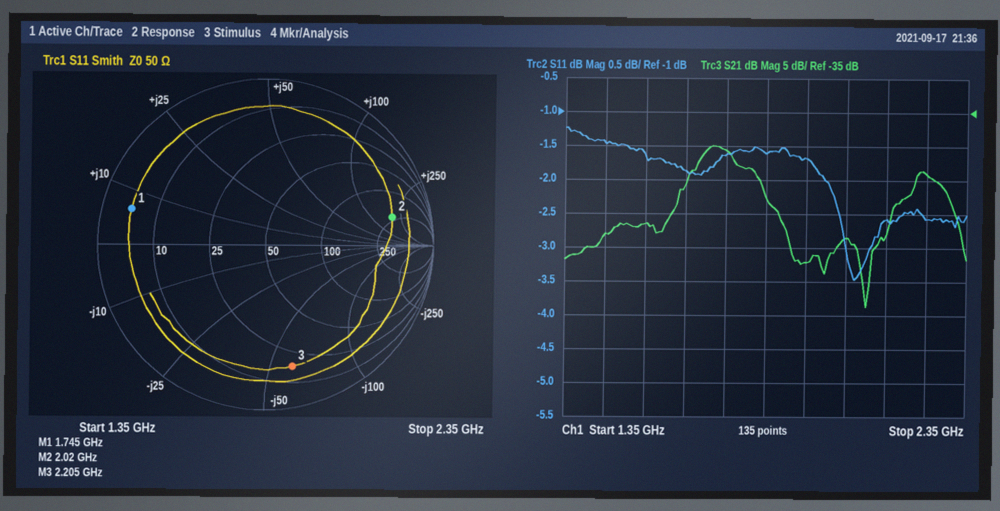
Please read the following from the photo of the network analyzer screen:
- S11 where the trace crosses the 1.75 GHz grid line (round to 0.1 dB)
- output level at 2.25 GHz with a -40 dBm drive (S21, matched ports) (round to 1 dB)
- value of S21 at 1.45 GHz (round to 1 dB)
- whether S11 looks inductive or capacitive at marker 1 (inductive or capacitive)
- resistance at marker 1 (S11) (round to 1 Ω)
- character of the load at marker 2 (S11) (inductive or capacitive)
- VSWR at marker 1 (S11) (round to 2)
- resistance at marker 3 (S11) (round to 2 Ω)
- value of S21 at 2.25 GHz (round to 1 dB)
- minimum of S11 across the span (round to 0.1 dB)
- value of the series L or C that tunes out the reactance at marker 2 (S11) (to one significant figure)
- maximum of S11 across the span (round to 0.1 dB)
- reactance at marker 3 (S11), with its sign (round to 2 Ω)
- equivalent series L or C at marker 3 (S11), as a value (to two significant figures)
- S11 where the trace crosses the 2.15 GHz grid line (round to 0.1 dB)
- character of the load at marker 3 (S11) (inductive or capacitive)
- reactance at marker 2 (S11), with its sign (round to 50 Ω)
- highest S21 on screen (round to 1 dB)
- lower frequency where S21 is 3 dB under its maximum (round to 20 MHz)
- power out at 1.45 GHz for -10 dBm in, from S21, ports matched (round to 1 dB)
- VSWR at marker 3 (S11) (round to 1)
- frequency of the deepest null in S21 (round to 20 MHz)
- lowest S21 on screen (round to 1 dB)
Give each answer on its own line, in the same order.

-1.6 dB
-84 dBm
-53 dB
inductive
5 Ω
inductive
10
18 Ω
-44 dB
-3.5 dB
400 fF
-1.2 dB
-60 Ω
1.2 pF
-2.6 dB
capacitive
+200 Ω
-40 dB
1.68 GHz
-63 dBm
7
2.10 GHz
-64 dB
